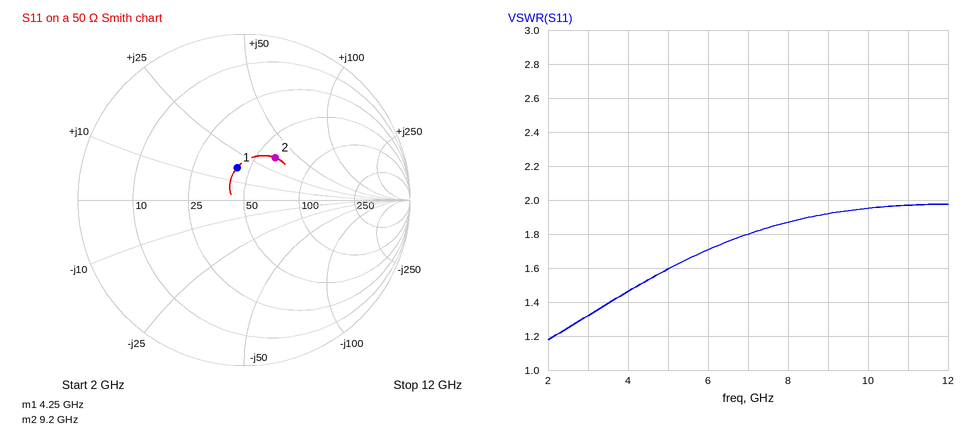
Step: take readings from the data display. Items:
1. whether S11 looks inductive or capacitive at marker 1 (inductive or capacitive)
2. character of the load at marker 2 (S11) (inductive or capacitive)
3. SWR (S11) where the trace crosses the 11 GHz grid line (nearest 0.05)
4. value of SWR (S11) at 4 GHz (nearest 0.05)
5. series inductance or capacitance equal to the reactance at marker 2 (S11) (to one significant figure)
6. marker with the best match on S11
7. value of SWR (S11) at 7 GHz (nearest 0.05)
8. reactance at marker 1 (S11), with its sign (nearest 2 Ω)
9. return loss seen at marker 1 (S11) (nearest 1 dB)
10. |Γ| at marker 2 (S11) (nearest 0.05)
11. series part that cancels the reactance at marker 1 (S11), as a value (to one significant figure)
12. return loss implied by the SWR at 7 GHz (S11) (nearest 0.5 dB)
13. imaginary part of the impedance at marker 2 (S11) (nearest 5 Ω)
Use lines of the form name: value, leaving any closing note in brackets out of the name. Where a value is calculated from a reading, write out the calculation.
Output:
whether S11 looks inductive or capacitive at marker 1: inductive
character of the load at marker 2 (S11): inductive
SWR (S11) where the trace crosses the 11 GHz grid line: 1.95
value of SWR (S11) at 4 GHz: 1.45
series inductance or capacitance equal to the reactance at marker 2 (S11): L = 35 Ω/(2π × 9.2 GHz) ≈ 605 pH, so 600 pH to one significant figure
marker with the best match on S11: marker 1
value of SWR (S11) at 7 GHz: 1.80
reactance at marker 1 (S11), with its sign: +18 Ω
return loss seen at marker 1 (S11): 14 dB
|Γ| at marker 2 (S11): 0.30
series part that cancels the reactance at marker 1 (S11), as a value: C = 1/(2π × 4.25 GHz × 18 Ω) ≈ 2 pF
return loss implied by the SWR at 7 GHz (S11): −20 log10((1.8 − 1)/(1.8 + 1)) ≈ 10.9 dB, so 11.0 dB to the nearest 0.5 dB
imaginary part of the impedance at marker 2 (S11): +35 Ω
